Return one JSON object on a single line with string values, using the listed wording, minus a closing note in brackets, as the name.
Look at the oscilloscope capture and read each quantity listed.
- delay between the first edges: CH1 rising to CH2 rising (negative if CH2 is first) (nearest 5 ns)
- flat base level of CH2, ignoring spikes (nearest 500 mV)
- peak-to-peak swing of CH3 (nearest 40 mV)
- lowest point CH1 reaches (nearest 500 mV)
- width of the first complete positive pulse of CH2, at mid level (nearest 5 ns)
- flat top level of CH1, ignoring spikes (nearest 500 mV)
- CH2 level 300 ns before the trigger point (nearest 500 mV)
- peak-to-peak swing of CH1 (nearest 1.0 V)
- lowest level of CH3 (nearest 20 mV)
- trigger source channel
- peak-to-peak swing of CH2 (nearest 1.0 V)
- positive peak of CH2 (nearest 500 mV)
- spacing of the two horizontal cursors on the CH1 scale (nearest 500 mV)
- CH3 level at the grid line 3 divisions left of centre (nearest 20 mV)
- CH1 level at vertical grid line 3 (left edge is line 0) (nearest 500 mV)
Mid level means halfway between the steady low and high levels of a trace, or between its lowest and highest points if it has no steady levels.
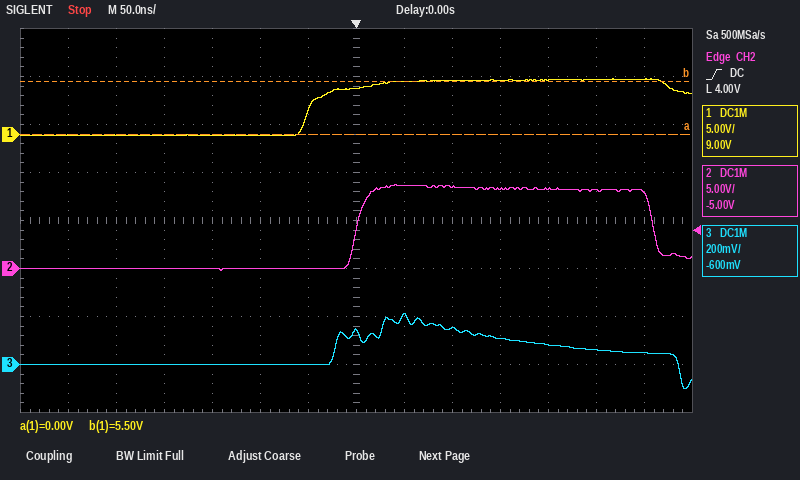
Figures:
{"delay between the first edges: CH1 rising to CH2 rising (negative if CH2 is first)": "+50 ns", "flat base level of CH2, ignoring spikes": "0.0 V", "peak-to-peak swing of CH3": "320 mV", "lowest point CH1 reaches": "0.0 V", "width of the first complete positive pulse of CH2, at mid level": "310 ns", "flat top level of CH1, ignoring spikes": "5.5 V", "CH2 level 300 ns before the trigger point": "0.0 V", "peak-to-peak swing of CH1": "6.0 V", "lowest level of CH3": "-100 mV", "trigger source channel": "CH2", "peak-to-peak swing of CH2": "9.0 V", "positive peak of CH2": "9.0 V", "spacing of the two horizontal cursors on the CH1 scale": "5.5 V", "CH3 level at the grid line 3 divisions left of centre": "0 mV", "CH1 level at vertical grid line 3 (left edge is line 0)": "0.0 V"}
